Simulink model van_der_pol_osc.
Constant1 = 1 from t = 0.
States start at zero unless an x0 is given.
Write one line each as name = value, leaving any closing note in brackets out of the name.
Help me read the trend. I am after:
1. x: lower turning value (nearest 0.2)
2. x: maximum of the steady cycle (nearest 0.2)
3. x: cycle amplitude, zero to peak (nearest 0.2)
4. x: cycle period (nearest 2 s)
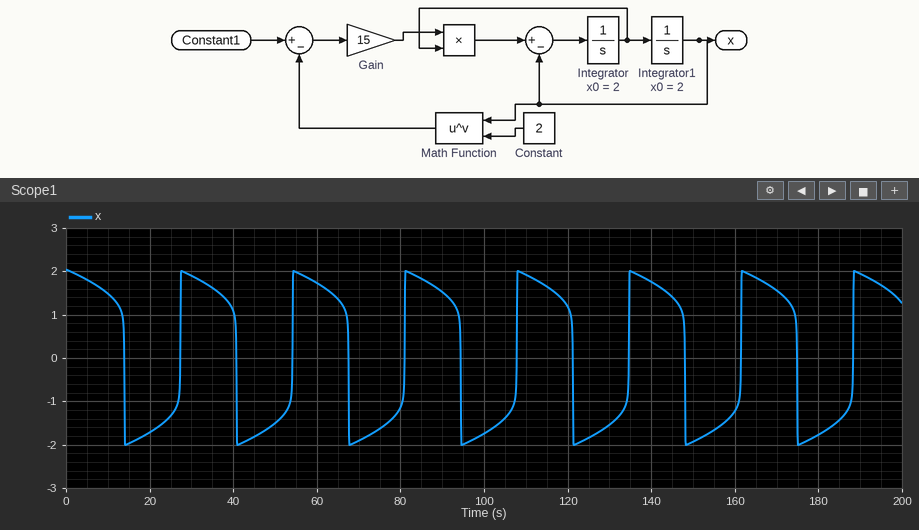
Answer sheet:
x: lower turning value = -2.0
x: maximum of the steady cycle = 2.0
x: cycle amplitude, zero to peak = 2.0
x: cycle period = 26 s
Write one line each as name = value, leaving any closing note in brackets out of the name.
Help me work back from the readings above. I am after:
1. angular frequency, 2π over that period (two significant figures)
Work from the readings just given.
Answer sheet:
angular frequency, 2π over that period = 0.24 rad/s
